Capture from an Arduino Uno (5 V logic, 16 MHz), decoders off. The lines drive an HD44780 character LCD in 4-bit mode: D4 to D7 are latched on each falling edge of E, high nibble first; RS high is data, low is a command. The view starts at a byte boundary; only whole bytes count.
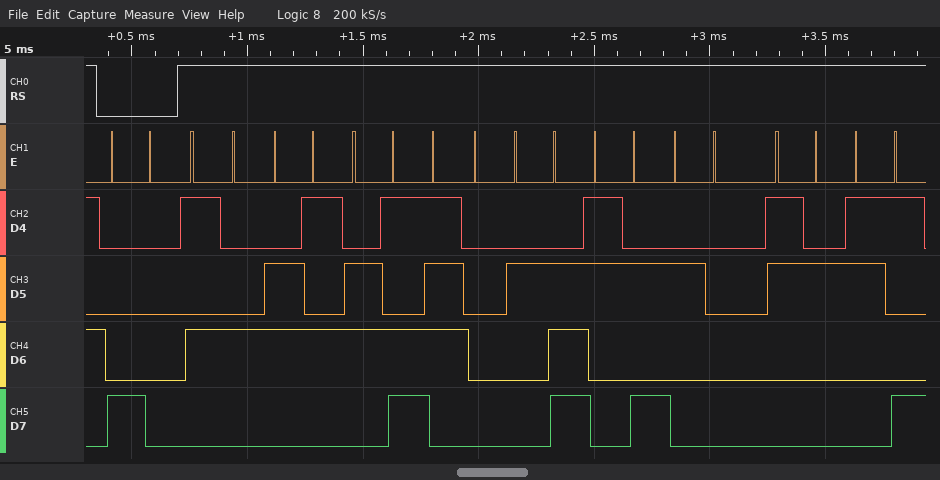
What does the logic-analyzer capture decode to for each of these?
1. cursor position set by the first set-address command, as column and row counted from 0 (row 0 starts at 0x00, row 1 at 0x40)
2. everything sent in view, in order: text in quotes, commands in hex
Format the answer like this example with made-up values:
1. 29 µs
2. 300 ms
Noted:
1. column 0, row 0
2. 0x80 "Temp.: 29"
